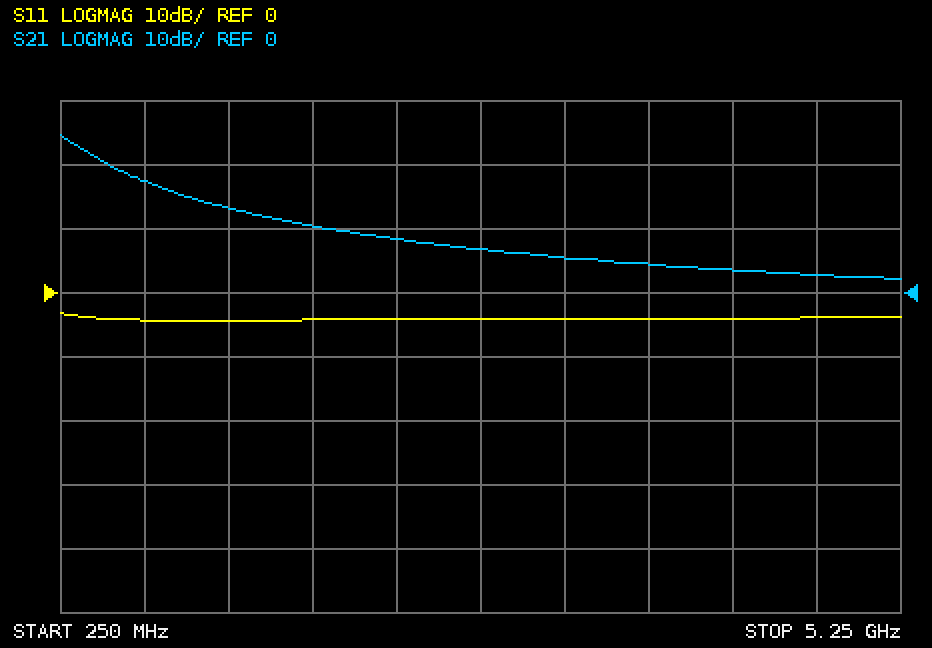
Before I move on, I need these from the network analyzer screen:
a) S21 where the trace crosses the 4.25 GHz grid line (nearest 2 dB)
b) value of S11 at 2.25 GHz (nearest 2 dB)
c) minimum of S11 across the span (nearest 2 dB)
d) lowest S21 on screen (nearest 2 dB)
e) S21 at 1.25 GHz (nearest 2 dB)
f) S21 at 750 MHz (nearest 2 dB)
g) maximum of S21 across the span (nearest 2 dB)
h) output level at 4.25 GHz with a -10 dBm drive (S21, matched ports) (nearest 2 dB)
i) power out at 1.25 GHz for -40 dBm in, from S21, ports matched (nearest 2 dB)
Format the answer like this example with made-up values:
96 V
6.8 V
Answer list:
4 dB
-4 dB
-4 dB
2 dB
14 dB
18 dB
24 dB
-6 dBm
-26 dBm
